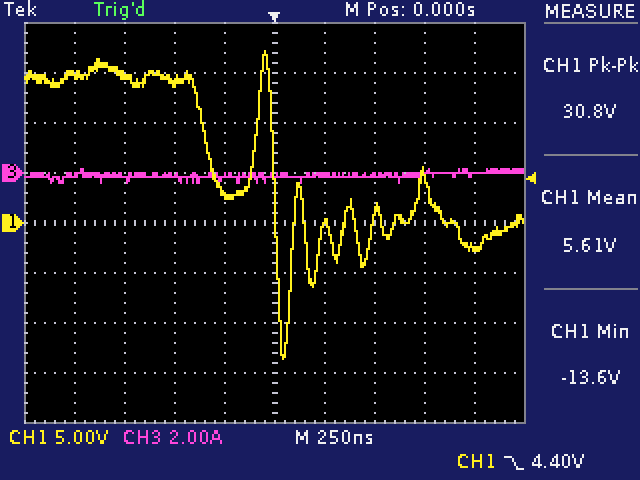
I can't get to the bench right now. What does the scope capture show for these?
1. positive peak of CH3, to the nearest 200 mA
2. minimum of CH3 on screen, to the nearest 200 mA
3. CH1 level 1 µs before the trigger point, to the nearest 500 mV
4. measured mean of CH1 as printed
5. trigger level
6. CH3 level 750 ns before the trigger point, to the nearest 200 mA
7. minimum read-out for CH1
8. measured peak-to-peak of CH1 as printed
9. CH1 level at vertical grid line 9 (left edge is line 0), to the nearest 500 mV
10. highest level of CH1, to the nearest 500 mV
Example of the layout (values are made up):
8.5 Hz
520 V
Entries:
200 mA
-400 mA
15.0 V
5.61 V
4.40 V
-200 mA
-13.6 V
30.8 V
-2.5 V
17.0 V
